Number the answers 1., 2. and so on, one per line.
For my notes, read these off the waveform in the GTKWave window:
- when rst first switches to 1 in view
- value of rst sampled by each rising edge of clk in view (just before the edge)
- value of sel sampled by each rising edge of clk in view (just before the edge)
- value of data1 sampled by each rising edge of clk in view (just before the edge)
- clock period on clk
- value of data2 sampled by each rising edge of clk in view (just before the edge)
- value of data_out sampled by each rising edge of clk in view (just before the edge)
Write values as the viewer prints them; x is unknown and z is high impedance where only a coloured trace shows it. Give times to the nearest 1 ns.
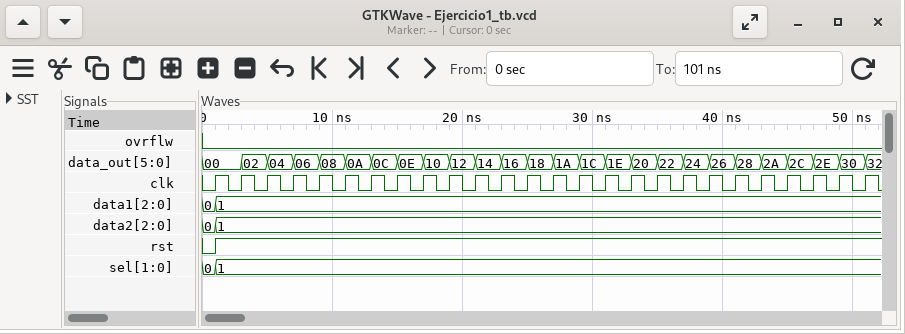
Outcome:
1. 1 ns
2. 0 1 1 1 1 1 1 1 1 1 1 1 1 1 1 1 1 1 1 1 1 1 1 1 1 1
3. 0, 1, 1, 1, 1, 1, 1, 1, 1, 1, 1, 1, 1, 1, 1, 1, 1, 1, 1, 1, 1, 1, 1, 1, 1, 1
4. 0, 1, 1, 1, 1, 1, 1, 1, 1, 1, 1, 1, 1, 1, 1, 1, 1, 1, 1, 1, 1, 1, 1, 1, 1, 1
5. 2 ns
6. 0, 1, 1, 1, 1, 1, 1, 1, 1, 1, 1, 1, 1, 1, 1, 1, 1, 1, 1, 1, 1, 1, 1, 1, 1, 1
7. 00, 00, 02, 04, 06, 08, 0A, 0C, 0E, 10, 12, 14, 16, 18, 1A, 1C, 1E, 20, 22, 24, 26, 28, 2A, 2C, 2E, 30
